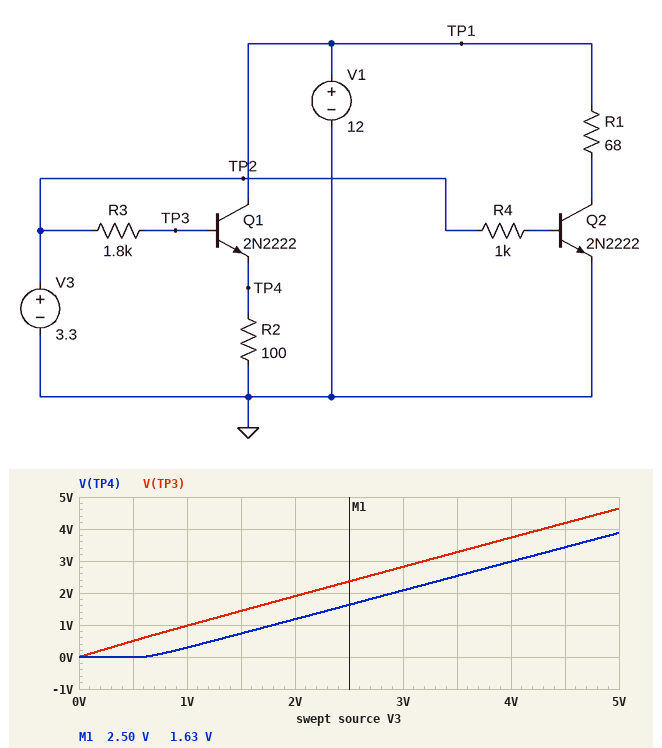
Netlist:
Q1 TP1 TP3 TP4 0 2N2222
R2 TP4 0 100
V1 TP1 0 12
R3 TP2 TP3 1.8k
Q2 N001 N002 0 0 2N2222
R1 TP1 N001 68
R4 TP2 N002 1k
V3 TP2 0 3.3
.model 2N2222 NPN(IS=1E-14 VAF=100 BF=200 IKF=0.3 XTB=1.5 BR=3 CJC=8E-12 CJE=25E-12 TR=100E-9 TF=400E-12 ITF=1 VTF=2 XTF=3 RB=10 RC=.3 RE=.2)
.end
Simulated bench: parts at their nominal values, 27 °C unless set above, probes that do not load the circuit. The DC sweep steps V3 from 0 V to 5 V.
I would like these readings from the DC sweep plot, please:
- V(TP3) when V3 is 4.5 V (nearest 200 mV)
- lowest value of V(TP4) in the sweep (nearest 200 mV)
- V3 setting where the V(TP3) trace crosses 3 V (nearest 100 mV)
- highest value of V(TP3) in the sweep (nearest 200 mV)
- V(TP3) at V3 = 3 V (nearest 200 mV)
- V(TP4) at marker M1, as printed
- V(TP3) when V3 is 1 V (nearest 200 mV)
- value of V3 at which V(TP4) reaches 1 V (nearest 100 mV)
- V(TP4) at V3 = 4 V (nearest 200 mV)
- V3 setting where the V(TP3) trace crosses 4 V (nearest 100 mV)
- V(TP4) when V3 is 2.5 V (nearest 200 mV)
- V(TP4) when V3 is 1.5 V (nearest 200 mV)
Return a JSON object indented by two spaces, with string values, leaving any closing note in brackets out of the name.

{
  "V(TP3) when V3 is 4.5 V": "4.2 V",
  "lowest value of V(TP4) in the sweep": "0 V",
  "V3 setting where the V(TP3) trace crosses 3 V": "3.2 V",
  "highest value of V(TP3) in the sweep": "4.6 V",
  "V(TP3) at V3 = 3 V": "2.8 V",
  "V(TP4) at marker M1, as printed": "1.63 V",
  "V(TP3) when V3 is 1 V": "1.0 V",
  "value of V3 at which V(TP4) reaches 1 V": "1.8 V",
  "V(TP4) at V3 = 4 V": "3.0 V",
  "V3 setting where the V(TP3) trace crosses 4 V": "4.3 V",
  "V(TP4) when V3 is 2.5 V": "1.6 V",
  "V(TP4) when V3 is 1.5 V": "800 mV"
}
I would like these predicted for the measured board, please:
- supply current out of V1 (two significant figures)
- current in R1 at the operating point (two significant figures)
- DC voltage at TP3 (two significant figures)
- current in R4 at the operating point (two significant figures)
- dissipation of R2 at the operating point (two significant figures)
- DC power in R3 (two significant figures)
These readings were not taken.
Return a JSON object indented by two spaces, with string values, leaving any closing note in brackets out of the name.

{
  "supply current out of V1": "200 mA",
  "current in R1 at the operating point": "170 mA",
  "DC voltage at TP3": "3.1 V",
  "current in R4 at the operating point": "2.4 mA",
  "dissipation of R2 at the operating point": "55 mW",
  "DC power in R3": "24 µW"
}
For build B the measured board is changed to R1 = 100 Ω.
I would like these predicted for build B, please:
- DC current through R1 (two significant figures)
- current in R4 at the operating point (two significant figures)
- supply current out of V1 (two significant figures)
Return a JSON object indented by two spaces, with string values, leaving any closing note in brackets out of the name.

{
  "DC current through R1": "120 mA",
  "current in R4 at the operating point": "2.5 mA",
  "supply current out of V1": "140 mA"
}
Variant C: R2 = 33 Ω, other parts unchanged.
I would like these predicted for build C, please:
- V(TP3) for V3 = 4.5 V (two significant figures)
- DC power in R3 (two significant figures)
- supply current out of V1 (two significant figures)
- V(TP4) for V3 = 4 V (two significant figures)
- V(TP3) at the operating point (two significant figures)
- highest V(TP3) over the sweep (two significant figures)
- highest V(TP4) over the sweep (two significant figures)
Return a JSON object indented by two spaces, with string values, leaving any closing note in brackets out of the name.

{
  "V(TP3) for V3 = 4.5 V": "3.6 V",
  "DC power in R3": "180 µW",
  "supply current out of V1": "230 mA",
  "V(TP4) for V3 = 4 V": "2.5 V",
  "V(TP3) at the operating point": "2.7 V",
  "highest V(TP3) over the sweep": "4.0 V",
  "highest V(TP4) over the sweep": "3.2 V"
}
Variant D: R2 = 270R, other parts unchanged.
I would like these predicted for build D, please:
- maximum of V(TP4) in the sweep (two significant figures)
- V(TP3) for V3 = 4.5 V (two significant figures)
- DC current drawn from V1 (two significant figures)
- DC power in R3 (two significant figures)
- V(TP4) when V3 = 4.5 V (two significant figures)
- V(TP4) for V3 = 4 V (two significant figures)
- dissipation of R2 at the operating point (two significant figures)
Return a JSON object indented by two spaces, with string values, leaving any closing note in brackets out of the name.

{
  "maximum of V(TP4) in the sweep": "4.1 V",
  "V(TP3) for V3 = 4.5 V": "4.4 V",
  "DC current drawn from V1": "180 mA",
  "DC power in R3": "3.4 µW",
  "V(TP4) when V3 = 4.5 V": "3.7 V",
  "V(TP4) for V3 = 4 V": "3.2 V",
  "dissipation of R2 at the operating point": "23 mW"
}
